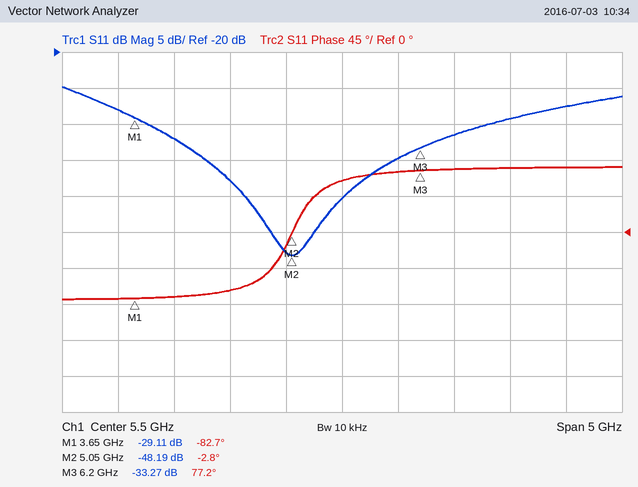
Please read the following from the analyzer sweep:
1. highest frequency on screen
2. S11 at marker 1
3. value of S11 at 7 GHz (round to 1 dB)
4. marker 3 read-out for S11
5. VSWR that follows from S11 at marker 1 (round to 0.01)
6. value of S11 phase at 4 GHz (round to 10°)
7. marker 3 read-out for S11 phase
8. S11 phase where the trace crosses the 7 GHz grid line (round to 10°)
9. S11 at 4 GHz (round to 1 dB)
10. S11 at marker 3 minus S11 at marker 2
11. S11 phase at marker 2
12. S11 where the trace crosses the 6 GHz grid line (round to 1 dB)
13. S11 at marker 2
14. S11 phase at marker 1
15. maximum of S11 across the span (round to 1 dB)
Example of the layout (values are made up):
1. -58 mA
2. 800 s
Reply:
1. 8 GHz
2. -29.11 dB
3. -29 dB
4. -33.27 dB
5. 1.07
6. -80°
7. 77.2°
8. 80°
9. -32 dB
10. 14.92 dB
11. -2.8°
12. -35 dB
13. -48.19 dB
14. -82.7°
15. -25 dB
